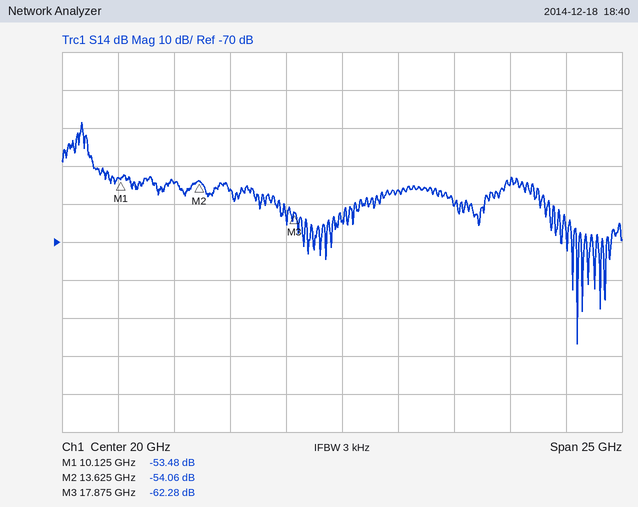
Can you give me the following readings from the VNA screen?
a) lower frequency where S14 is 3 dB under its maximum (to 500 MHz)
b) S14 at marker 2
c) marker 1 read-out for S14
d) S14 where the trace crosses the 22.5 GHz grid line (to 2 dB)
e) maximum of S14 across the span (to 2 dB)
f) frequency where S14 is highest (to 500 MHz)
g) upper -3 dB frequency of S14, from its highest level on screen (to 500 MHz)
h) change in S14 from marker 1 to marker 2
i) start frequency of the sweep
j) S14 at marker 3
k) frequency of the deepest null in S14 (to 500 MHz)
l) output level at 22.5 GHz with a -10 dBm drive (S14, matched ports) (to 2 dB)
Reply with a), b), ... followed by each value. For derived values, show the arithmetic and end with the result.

a) 8.5 GHz
b) -54.06 dB
c) -53.48 dB
d) -56 dB
e) -38 dB
f) 8.5 GHz
g) 8.5 GHz
h) -54.06 − (-53.48) = -0.58 dB
i) 7.5 GHz
j) -62.28 dB
k) 30.5 GHz
l) -10 dBm + (-56 dB) = -66 dBm
